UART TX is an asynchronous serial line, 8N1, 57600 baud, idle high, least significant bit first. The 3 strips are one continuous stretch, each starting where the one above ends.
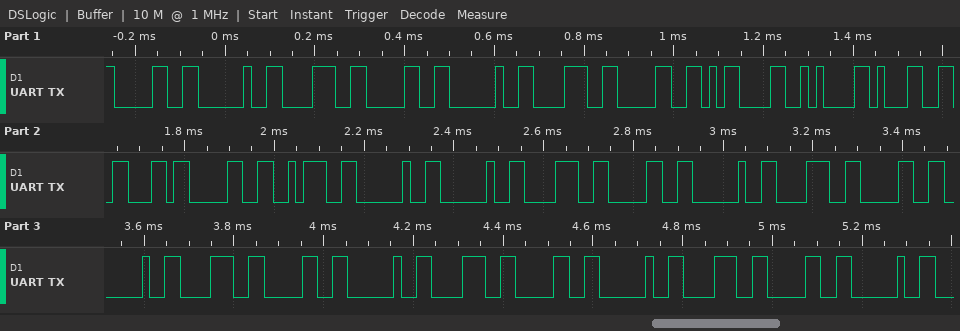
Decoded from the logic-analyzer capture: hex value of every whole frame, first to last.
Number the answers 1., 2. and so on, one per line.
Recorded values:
1. 30 20 38 30 20 38 30 0D 0A 31 63 30 3A 20 20 38 30 20 38 30 20 38 30 20 38 30 20 38 30 20
